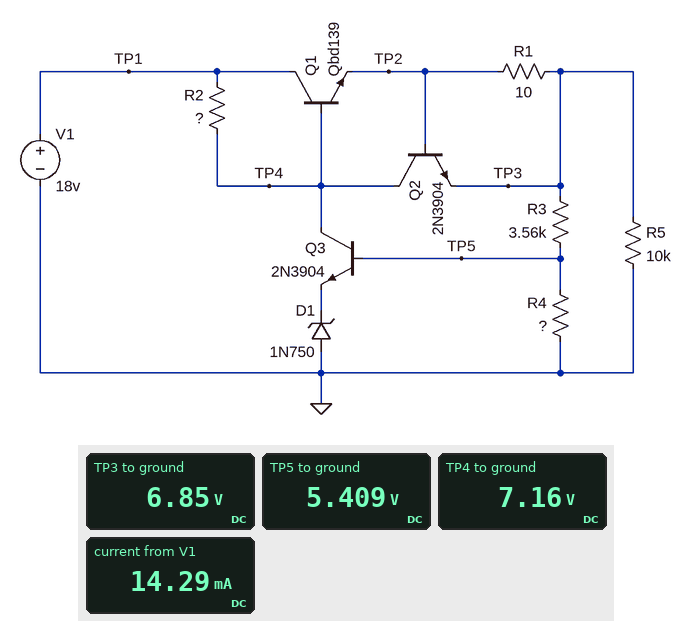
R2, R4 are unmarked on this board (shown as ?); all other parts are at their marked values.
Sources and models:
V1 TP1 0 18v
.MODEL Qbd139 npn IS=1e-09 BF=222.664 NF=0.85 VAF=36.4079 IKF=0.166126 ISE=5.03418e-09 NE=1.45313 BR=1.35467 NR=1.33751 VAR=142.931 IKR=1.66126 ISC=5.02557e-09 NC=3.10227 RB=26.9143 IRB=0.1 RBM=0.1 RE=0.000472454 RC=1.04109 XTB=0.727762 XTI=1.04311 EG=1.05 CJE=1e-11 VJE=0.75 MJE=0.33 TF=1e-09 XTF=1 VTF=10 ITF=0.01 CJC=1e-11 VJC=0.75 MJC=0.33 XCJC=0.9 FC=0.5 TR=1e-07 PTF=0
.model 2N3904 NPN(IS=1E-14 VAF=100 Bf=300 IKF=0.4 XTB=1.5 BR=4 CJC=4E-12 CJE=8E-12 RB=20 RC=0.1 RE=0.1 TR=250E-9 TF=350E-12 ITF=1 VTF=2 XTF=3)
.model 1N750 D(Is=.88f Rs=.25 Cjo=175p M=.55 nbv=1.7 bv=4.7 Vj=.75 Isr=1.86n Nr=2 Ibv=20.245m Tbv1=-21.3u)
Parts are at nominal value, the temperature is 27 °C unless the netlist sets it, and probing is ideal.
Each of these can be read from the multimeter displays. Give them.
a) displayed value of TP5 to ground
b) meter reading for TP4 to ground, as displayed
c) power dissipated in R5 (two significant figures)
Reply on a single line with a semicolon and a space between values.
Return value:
5.409 V; 7.16 V; 4.7 mW
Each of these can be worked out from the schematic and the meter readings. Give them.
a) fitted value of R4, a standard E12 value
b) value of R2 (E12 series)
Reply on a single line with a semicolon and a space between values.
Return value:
15 kΩ; 820 Ω
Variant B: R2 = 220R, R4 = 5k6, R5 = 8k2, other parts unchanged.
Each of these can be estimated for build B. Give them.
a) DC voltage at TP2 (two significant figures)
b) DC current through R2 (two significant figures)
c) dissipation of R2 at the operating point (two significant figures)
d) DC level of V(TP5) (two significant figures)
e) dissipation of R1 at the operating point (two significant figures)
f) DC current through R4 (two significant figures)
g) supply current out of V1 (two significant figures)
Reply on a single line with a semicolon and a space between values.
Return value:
9.5 V; 37 mA; 310 mW; 5.5 V; 51 µW; 980 µA; 40 mA
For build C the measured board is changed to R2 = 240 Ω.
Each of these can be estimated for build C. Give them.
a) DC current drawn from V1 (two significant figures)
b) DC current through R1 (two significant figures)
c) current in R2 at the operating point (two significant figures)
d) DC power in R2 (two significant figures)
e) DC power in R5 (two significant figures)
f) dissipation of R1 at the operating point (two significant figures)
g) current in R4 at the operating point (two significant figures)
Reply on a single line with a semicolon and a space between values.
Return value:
44 mA; 1.3 mA; 43 mA; 440 mW; 5.4 mW; 16 µW; 370 µA
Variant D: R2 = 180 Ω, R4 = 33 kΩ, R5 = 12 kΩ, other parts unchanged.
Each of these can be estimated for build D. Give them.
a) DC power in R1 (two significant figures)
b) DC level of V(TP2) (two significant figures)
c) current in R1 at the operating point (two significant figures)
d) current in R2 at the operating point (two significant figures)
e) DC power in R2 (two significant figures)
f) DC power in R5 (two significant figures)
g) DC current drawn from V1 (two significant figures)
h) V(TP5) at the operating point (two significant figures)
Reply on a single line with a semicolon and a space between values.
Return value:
9.4 µW; 6.9 V; 970 µA; 60 mA; 640 mW; 4.0 mW; 61 mA; 5.5 V
